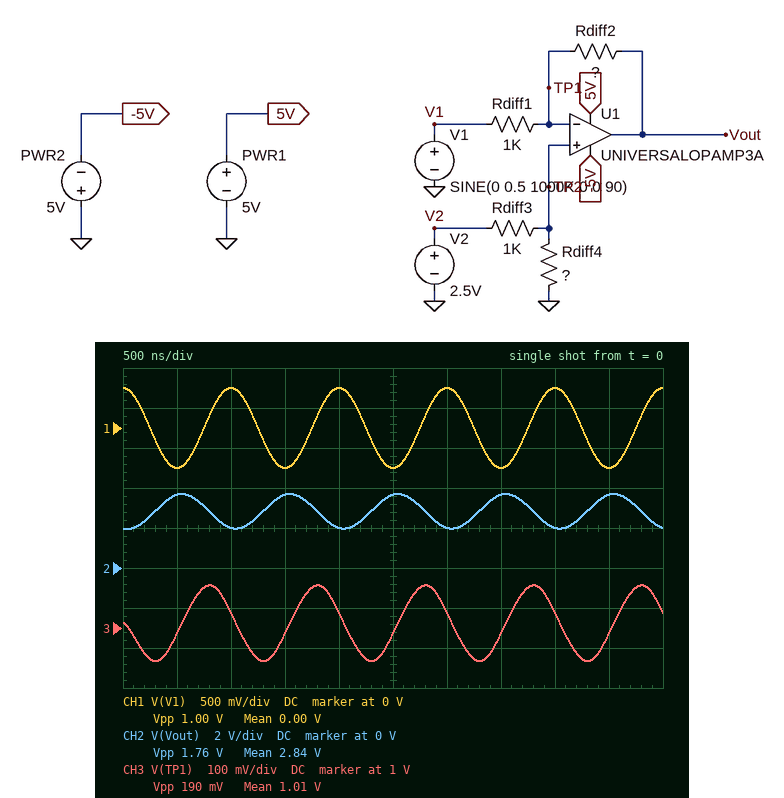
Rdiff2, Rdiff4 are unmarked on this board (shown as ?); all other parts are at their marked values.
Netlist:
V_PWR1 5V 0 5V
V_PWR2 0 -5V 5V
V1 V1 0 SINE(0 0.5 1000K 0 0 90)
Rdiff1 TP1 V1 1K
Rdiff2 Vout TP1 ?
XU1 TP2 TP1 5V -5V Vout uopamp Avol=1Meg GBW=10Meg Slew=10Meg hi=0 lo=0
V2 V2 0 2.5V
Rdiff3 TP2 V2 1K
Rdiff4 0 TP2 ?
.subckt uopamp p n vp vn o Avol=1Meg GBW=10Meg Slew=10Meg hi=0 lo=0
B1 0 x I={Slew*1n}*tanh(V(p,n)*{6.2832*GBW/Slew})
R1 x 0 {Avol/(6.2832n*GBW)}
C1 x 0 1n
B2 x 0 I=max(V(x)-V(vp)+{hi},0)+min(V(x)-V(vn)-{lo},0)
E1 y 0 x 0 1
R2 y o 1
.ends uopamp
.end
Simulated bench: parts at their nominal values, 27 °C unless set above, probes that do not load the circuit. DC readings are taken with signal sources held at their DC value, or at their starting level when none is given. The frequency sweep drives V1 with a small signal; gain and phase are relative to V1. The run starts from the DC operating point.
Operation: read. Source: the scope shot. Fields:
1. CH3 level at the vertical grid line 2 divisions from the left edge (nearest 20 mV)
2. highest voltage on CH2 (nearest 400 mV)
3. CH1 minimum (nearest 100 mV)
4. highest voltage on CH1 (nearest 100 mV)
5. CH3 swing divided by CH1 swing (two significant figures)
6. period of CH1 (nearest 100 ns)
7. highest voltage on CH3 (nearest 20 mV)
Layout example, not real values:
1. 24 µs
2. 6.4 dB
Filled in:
1. 1.04 V
2. 3.6 V
3. -500 mV
4. 500 mV
5. 0.19
6. 1.0 µs
7. 1.10 V
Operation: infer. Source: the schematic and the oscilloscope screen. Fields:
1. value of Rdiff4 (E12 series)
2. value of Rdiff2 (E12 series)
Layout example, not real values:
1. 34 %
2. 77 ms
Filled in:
1. 680 Ω
2. 1.8 kΩ
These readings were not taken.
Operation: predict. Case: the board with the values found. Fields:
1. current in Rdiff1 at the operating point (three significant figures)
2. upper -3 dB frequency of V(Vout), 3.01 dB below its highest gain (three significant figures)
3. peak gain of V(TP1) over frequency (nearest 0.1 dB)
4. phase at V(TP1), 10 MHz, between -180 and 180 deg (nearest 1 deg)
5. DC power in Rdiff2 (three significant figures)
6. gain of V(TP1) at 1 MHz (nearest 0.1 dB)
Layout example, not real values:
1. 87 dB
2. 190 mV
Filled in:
1. 512 µA
2. 3.57 MHz
3. -3.8 dB
4. 20 deg
5. 472 µW
6. -15.2 dB
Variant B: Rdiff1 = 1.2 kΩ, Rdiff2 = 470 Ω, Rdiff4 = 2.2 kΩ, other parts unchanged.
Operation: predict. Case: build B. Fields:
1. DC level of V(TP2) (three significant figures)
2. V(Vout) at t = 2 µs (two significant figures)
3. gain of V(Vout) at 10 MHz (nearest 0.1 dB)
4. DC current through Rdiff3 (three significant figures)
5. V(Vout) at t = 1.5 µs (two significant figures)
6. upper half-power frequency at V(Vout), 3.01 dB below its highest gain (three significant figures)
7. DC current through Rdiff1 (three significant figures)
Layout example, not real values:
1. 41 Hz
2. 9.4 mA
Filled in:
1. 1.72 V
2. 2.2 V
3. -12.8 dB
4. 781 µA
5. 2.6 V
6. 7.18 MHz
7. 1.02 mA
